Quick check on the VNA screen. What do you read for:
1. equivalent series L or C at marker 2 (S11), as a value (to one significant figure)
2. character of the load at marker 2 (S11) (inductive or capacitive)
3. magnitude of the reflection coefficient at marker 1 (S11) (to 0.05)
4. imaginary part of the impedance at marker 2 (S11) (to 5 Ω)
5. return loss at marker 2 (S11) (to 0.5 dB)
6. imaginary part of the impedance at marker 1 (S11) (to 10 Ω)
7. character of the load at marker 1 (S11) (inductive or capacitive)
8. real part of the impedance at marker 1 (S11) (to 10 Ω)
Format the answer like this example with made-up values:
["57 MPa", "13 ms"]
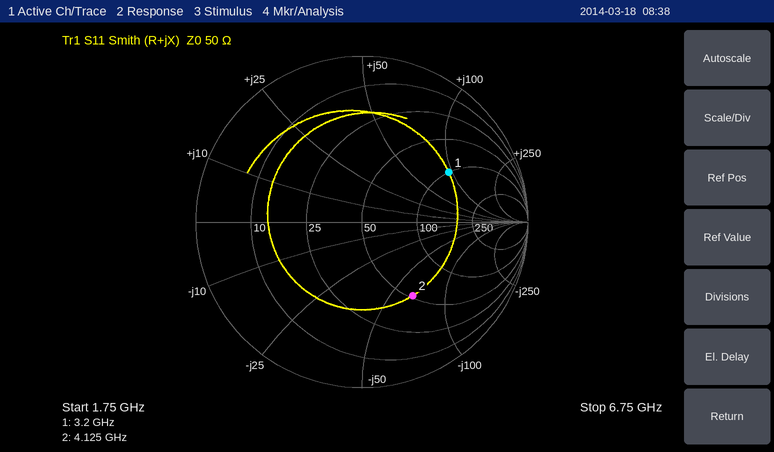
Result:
["600 fF", "capacitive", "0.60", "-65 Ω", "5.5 dB", "+90 Ω", "inductive", "100 Ω"]
